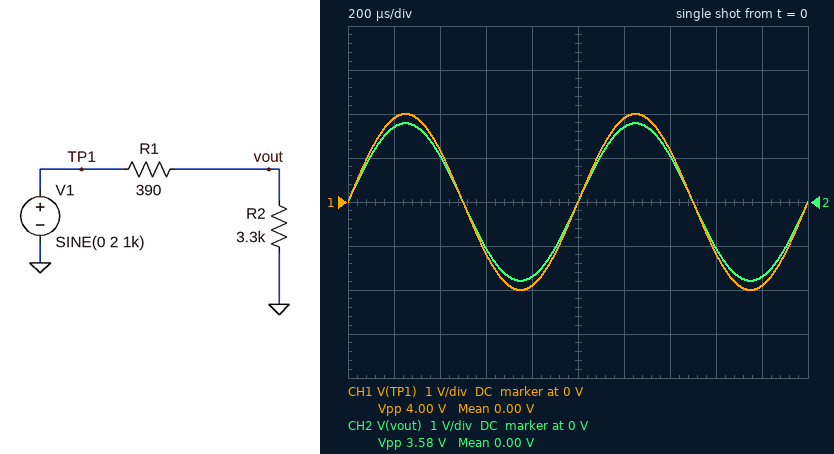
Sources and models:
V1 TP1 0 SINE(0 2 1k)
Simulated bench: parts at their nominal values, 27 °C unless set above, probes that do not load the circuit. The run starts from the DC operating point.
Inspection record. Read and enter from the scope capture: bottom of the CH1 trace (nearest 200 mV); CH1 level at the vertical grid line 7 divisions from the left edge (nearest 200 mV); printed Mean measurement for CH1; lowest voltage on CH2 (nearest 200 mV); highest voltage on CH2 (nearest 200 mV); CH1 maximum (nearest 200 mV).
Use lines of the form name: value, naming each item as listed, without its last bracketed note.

bottom of the CH1 trace: -2.0 V
CH1 level at the vertical grid line 7 divisions from the left edge: 1.2 V
printed Mean measurement for CH1: 0.00 V
lowest voltage on CH2: -1.8 V
highest voltage on CH2: 1.8 V
CH1 maximum: 2.0 V
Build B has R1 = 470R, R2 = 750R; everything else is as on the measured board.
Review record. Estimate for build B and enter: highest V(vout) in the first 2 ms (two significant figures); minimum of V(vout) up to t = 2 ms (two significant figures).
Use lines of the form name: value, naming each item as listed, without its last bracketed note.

highest V(vout) in the first 2 ms: 1.2 V
minimum of V(vout) up to t = 2 ms: -1.2 V
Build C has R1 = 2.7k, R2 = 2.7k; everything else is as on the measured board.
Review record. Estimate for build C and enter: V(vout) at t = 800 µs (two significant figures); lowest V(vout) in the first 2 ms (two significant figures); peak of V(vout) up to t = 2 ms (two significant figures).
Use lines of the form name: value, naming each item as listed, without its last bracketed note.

V(vout) at t = 800 µs: -950 mV
lowest V(vout) in the first 2 ms: -1.0 V
peak of V(vout) up to t = 2 ms: 1.0 V
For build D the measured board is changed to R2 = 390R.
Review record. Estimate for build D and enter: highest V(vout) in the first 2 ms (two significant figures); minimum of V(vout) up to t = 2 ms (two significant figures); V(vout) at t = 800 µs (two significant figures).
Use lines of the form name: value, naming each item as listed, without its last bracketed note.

highest V(vout) in the first 2 ms: 1.0 V
minimum of V(vout) up to t = 2 ms: -1.0 V
V(vout) at t = 800 µs: -950 mV
